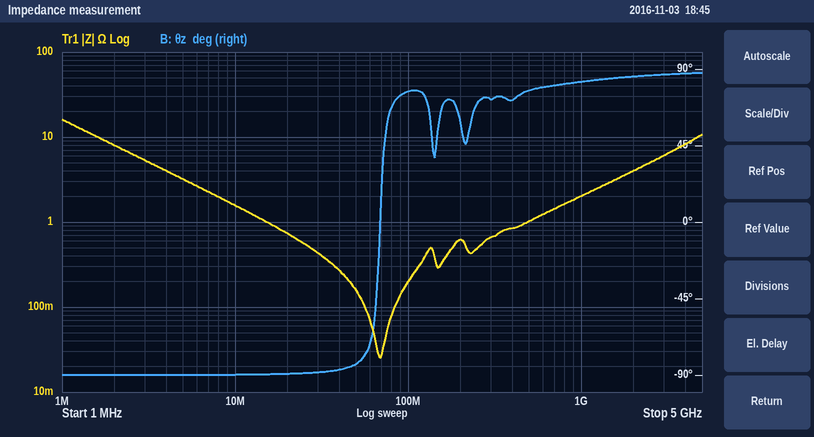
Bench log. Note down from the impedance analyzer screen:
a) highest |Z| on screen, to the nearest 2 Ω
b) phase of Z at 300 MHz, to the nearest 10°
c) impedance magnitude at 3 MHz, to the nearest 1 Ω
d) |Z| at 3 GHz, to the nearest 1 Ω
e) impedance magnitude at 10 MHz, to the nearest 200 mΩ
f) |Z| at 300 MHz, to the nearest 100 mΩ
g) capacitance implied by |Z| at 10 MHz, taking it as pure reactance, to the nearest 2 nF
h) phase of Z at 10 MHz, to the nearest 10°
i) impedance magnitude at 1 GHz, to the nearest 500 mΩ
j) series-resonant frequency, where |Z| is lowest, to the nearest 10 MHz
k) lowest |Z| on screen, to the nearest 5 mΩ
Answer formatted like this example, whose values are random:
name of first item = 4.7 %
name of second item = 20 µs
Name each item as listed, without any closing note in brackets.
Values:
highest |Z| on screen, to the nearest 2 Ω = 16 Ω
phase of Z at 300 MHz, to the nearest 10° = 70°
impedance magnitude at 3 MHz, to the nearest 1 Ω = 5 Ω
|Z| at 3 GHz, to the nearest 1 Ω = 6 Ω
impedance magnitude at 10 MHz, to the nearest 200 mΩ = 1.6 Ω
|Z| at 300 MHz, to the nearest 100 mΩ = 700 mΩ
capacitance implied by |Z| at 10 MHz, taking it as pure reactance, to the nearest 2 nF = 10 nF
phase of Z at 10 MHz, to the nearest 10° = -90°
impedance magnitude at 1 GHz, to the nearest 500 mΩ = 2.0 Ω
series-resonant frequency, where |Z| is lowest, to the nearest 10 MHz = 70 MHz
lowest |Z| on screen, to the nearest 5 mΩ = 25 mΩ
